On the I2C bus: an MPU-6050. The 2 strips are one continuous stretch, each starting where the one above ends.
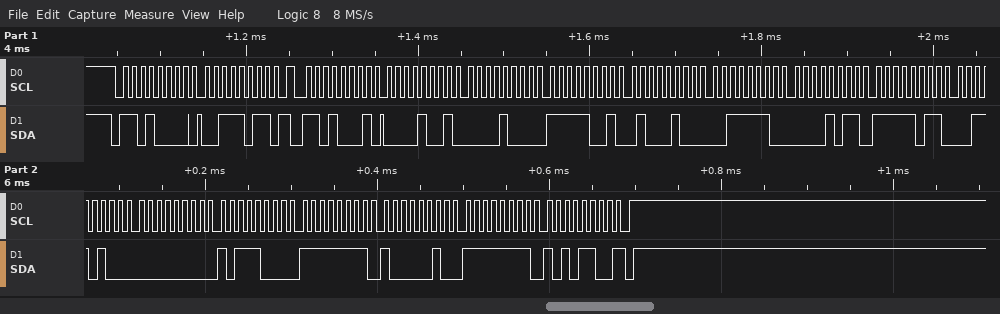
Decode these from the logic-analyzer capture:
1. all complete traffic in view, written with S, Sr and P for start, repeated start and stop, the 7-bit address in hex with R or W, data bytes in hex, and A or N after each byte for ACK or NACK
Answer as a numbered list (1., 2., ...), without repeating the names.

1. S 68W A 3B A Sr 68R A 09 A 08 A F9 A 44 A 3E A 0B A FB A 34 A 00 A B8 A FF A 82 A FF A AC N P
